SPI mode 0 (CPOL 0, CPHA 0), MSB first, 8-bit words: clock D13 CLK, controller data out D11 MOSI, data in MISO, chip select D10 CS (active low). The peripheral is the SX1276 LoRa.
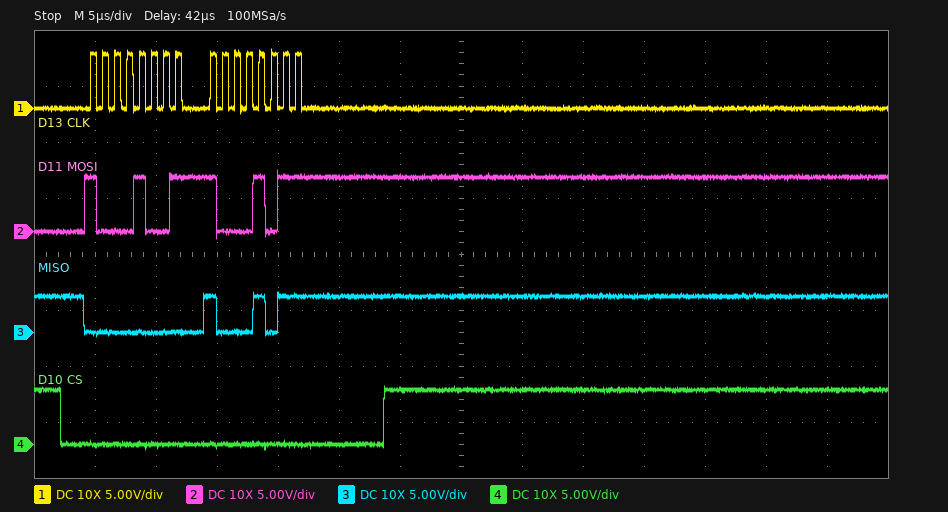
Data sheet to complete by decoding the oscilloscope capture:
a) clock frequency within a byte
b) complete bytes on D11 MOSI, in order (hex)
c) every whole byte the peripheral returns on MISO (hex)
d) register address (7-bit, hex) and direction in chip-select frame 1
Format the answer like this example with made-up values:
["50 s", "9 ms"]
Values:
["1 MHz", "0x89 0x8B", "0x00 0x8B", "0x09 write"]
